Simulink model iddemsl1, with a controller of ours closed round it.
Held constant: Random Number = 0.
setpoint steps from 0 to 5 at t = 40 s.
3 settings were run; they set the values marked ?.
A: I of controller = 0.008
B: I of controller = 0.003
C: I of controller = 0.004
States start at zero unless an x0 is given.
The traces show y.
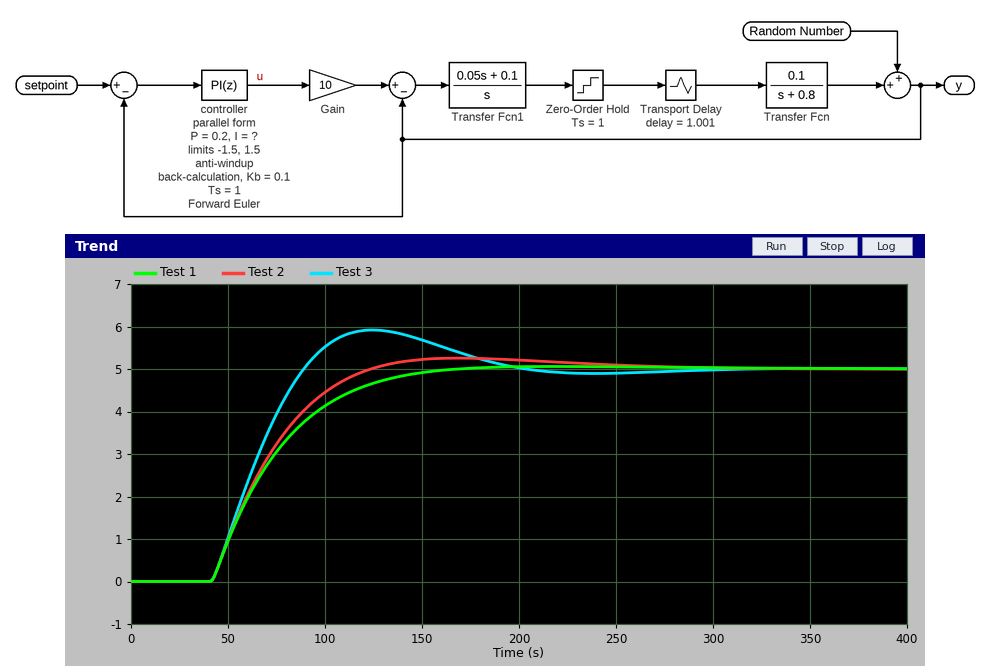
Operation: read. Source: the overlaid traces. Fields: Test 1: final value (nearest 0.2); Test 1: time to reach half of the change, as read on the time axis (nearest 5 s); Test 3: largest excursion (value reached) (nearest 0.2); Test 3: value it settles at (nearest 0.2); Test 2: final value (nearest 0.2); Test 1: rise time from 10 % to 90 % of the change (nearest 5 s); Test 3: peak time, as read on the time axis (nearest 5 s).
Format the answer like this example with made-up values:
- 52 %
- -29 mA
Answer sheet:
- 5.0
- 65 s
- 6.0
- 5.0
- 5.0
- 70 s
- 125 s
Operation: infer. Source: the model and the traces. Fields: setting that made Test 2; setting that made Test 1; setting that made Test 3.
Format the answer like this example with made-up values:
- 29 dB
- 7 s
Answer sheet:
- C
- B
- A
